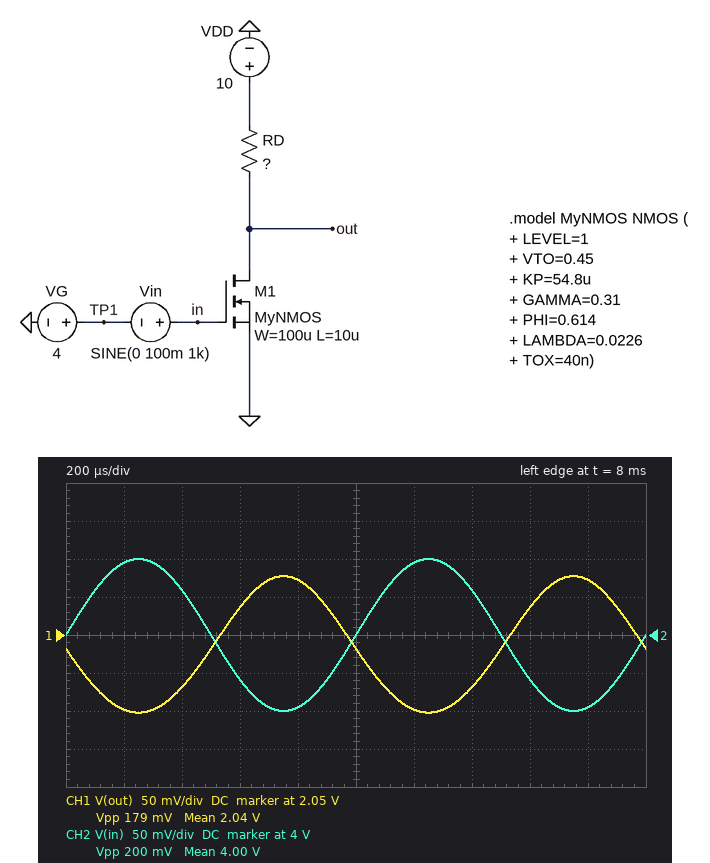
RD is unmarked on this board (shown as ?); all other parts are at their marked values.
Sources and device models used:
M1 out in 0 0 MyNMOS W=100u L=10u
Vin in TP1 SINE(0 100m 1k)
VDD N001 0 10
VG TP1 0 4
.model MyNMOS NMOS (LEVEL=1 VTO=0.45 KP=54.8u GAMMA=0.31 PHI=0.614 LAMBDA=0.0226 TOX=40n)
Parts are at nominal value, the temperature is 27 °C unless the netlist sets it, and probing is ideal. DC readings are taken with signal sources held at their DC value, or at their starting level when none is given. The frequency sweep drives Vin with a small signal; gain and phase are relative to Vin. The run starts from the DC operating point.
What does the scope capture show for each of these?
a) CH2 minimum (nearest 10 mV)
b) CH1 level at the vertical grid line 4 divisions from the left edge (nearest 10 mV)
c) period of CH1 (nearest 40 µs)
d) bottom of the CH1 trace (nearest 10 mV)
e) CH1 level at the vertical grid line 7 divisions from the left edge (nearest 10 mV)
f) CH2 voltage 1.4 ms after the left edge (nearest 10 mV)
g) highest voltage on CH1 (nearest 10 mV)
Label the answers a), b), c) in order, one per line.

a) 3.90 V
b) 2.12 V
c) 1.00 ms
d) 1.95 V
e) 1.98 V
f) 4.06 V
g) 2.13 V
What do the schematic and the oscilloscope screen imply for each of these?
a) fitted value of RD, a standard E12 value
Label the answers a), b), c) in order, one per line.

a) 2.7 kΩ
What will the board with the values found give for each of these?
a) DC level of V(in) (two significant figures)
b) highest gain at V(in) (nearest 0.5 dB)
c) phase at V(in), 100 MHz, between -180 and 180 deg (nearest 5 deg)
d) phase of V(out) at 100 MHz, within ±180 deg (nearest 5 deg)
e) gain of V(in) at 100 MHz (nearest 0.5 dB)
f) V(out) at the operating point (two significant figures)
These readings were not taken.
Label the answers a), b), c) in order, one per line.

a) 4.0 V
b) 0 dB
c) 0 deg
d) 165 deg
e) 0 dB
f) 2.0 V
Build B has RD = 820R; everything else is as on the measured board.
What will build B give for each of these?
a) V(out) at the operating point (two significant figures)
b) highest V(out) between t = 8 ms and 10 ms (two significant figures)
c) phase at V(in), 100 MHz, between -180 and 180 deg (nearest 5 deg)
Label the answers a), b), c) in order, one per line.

a) 6.7 V
b) 6.9 V
c) 0 deg
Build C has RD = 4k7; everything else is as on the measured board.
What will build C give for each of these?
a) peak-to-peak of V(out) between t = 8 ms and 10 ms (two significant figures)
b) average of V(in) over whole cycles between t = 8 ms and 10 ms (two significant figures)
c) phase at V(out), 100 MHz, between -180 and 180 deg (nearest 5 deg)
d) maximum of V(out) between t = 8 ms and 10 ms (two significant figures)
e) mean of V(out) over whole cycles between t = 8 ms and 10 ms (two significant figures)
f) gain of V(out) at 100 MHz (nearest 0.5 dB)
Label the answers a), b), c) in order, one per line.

a) 78 mV
b) 4.0 V
c) 150 deg
d) 1.2 V
e) 1.1 V
f) -7.5 dB
